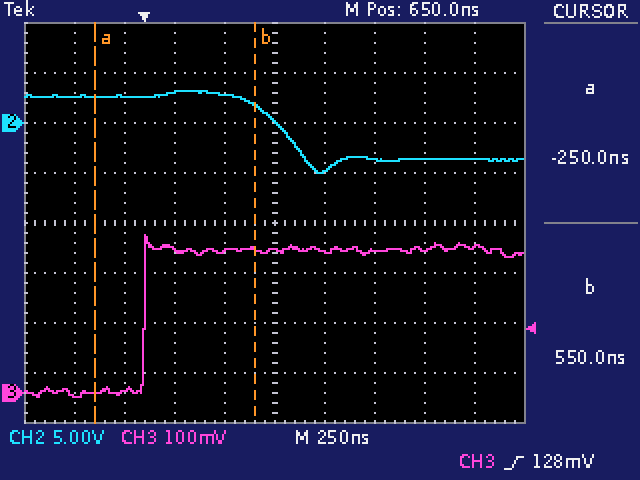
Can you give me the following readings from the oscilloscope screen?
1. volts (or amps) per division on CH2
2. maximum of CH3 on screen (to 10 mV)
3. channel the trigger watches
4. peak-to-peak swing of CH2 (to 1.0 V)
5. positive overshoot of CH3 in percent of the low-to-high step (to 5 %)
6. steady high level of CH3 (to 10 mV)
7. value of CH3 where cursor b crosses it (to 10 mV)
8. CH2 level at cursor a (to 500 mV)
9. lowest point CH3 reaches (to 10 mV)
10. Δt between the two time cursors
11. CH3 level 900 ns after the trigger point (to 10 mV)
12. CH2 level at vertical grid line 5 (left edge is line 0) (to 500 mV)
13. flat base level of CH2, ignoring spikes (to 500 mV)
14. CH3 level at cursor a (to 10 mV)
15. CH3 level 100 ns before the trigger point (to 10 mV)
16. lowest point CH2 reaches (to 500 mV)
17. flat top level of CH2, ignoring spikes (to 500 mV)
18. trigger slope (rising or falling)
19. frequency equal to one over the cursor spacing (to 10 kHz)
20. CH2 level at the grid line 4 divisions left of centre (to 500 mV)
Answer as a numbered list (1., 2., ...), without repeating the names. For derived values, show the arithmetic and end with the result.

1. 5 V
2. 320 mV
3. CH3
4. 8.0 V
5. 10 %
6. 290 mV
7. 290 mV
8. 2.5 V
9. -10 mV
10. 550 ns − (-250 ns) = 800 ns
11. 280 mV
12. 0.0 V
13. -3.5 V
14. 0 mV
15. 0 mV
16. -5.0 V
17. 2.5 V
18. rising
19. 1 / 800 ns ≈ 1.25 MHz
20. 2.5 V
